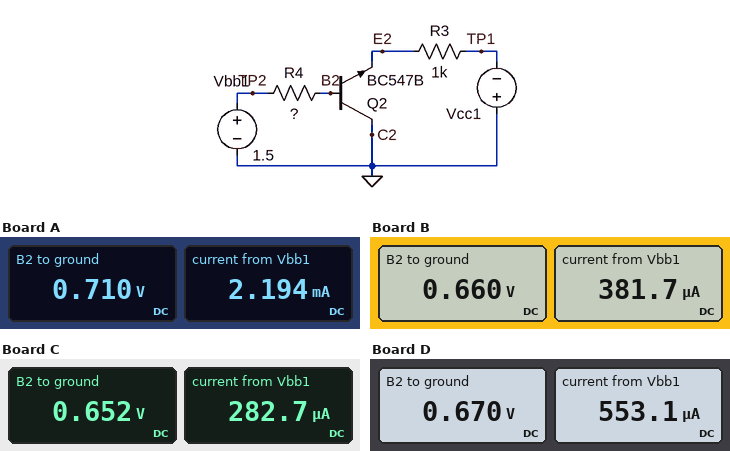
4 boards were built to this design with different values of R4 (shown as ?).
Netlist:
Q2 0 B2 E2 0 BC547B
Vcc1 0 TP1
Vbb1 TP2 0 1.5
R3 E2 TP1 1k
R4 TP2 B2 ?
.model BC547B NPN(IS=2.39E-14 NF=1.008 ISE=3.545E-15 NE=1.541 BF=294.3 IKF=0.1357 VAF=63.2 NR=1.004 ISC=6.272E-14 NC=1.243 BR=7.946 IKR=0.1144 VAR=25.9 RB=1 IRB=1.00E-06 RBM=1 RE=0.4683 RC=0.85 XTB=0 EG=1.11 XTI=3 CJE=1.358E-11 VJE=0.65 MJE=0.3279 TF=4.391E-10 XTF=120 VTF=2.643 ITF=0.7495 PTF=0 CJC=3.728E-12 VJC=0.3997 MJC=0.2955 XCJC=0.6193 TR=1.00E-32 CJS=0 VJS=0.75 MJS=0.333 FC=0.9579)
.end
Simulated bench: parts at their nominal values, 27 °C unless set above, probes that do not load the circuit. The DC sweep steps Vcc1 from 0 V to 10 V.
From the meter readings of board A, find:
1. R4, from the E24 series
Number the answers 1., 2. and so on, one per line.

1. 360 Ω
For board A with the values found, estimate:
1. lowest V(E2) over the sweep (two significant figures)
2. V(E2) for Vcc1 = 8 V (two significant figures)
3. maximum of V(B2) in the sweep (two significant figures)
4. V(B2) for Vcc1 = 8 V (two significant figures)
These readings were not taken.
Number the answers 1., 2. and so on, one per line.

1. -30 mV
2. -25 mV
3. 710 mV
4. 700 mV
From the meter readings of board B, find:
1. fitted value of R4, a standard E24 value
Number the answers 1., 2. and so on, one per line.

1. 2.2 kΩ
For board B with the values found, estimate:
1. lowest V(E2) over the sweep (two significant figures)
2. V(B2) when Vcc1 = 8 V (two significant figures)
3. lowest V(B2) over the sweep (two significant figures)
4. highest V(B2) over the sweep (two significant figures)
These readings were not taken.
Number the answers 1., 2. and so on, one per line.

1. -62 mV
2. 650 mV
3. 650 mV
4. 660 mV
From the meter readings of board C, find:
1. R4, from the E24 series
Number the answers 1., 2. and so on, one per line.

1. 3 kΩ
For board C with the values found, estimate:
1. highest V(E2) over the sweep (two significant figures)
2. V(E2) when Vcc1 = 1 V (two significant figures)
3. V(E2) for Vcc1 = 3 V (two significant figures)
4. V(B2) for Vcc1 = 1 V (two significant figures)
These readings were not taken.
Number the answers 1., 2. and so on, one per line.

1. -2.2 mV
2. -15 mV
3. -33 mV
4. 650 mV
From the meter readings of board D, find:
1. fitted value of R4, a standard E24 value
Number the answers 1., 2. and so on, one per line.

1. 1.5 kΩ
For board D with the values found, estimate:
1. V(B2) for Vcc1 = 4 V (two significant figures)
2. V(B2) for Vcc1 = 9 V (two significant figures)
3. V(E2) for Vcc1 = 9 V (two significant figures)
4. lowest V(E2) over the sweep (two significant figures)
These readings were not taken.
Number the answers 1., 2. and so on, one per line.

1. 670 mV
2. 660 mV
3. -50 mV
4. -53 mV
